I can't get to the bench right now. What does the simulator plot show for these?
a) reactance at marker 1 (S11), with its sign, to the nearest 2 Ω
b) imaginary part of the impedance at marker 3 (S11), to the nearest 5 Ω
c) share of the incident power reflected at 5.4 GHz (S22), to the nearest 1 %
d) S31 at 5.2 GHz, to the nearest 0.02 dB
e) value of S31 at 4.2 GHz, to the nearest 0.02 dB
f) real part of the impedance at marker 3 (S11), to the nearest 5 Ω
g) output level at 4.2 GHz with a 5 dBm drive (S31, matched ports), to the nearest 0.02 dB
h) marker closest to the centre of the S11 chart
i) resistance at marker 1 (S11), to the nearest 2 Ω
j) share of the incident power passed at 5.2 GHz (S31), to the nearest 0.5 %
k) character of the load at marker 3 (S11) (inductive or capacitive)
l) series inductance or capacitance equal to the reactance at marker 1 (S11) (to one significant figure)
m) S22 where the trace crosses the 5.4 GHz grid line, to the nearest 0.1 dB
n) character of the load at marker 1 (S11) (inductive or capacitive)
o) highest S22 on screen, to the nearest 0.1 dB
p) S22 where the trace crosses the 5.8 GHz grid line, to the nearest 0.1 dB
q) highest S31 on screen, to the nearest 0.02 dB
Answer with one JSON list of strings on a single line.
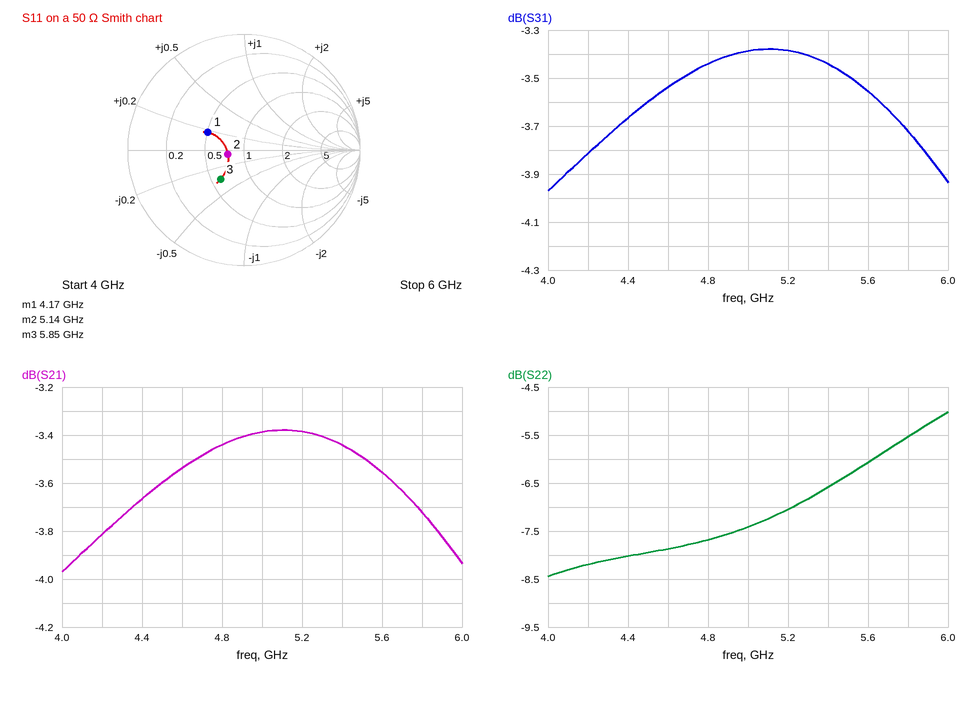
["+8 Ω", "-15 Ω", "22 %", "-3.38 dB", "-3.82 dB", "30 Ω", "1.18 dBm", "marker 2", "26 Ω", "46.0 %", "capacitive", "300 pH", "-6.6 dB", "inductive", "-5.0 dB", "-5.5 dB", "-3.38 dB"]
